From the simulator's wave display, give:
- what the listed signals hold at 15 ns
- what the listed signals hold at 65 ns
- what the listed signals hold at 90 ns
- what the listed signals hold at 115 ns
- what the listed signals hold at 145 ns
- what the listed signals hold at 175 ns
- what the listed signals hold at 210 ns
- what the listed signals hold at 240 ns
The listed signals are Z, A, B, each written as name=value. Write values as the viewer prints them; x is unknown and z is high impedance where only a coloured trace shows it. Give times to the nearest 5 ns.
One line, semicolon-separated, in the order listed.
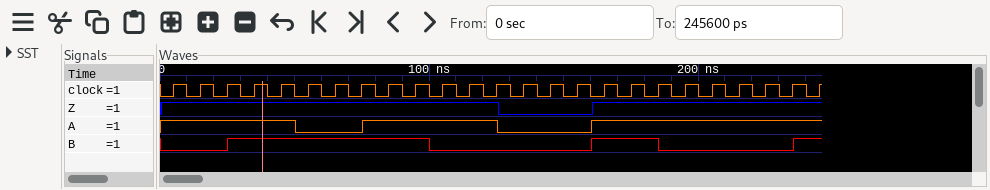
Z=1, A=1, B=0; Z=1, A=0, B=1; Z=1, A=1, B=1; Z=1, A=1, B=0; Z=0, A=0, B=0; Z=1, A=1, B=1; Z=1, A=1, B=0; Z=1, A=1, B=1
